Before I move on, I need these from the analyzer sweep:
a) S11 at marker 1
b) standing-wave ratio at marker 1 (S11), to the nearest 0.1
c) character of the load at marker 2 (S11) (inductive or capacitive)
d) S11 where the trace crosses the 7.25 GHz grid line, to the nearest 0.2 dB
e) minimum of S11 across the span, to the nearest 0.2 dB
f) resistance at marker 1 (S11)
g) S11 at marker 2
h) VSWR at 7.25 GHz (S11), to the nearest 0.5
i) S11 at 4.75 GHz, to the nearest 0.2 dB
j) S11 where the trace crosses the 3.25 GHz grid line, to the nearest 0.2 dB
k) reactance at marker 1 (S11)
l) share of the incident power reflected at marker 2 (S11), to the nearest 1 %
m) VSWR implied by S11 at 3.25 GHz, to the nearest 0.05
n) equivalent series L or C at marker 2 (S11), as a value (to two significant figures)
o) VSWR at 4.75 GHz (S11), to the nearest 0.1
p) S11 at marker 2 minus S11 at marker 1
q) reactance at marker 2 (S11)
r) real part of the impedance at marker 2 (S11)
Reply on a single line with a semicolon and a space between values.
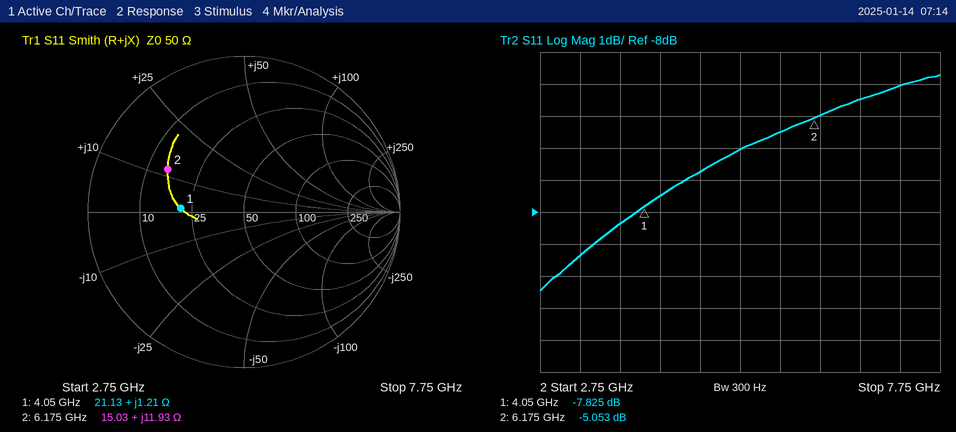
-7.825 dB; 2.4; inductive; -4.0 dB; -10.4 dB; 21.13 Ω; -5.053 dB; 4.5; -6.8 dB; -9.4 dB; +1.21 Ω; 31 %; 2.05; 310 pH; 2.7; 2.772 dB; +11.93 Ω; 15.03 Ω
